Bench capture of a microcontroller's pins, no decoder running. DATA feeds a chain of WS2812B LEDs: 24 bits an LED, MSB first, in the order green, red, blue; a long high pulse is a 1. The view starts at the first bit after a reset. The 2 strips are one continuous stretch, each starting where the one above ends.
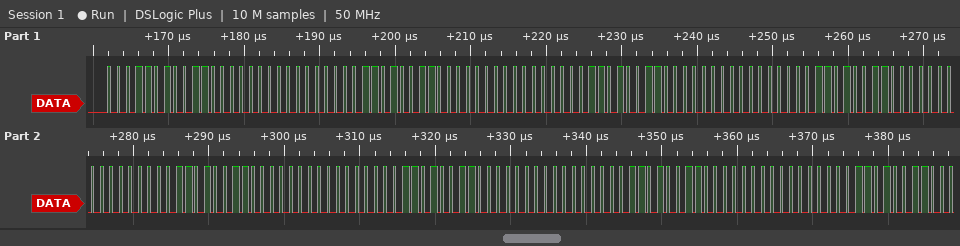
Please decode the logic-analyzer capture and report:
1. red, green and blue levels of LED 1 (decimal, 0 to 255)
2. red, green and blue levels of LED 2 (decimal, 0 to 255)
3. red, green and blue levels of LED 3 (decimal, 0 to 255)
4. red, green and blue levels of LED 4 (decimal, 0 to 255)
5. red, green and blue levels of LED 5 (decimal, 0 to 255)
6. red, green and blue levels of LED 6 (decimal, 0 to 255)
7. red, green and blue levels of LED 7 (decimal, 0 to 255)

96, 26, 0
96, 26, 0
96, 26, 0
96, 26, 0
96, 26, 0
96, 26, 0
96, 26, 0
